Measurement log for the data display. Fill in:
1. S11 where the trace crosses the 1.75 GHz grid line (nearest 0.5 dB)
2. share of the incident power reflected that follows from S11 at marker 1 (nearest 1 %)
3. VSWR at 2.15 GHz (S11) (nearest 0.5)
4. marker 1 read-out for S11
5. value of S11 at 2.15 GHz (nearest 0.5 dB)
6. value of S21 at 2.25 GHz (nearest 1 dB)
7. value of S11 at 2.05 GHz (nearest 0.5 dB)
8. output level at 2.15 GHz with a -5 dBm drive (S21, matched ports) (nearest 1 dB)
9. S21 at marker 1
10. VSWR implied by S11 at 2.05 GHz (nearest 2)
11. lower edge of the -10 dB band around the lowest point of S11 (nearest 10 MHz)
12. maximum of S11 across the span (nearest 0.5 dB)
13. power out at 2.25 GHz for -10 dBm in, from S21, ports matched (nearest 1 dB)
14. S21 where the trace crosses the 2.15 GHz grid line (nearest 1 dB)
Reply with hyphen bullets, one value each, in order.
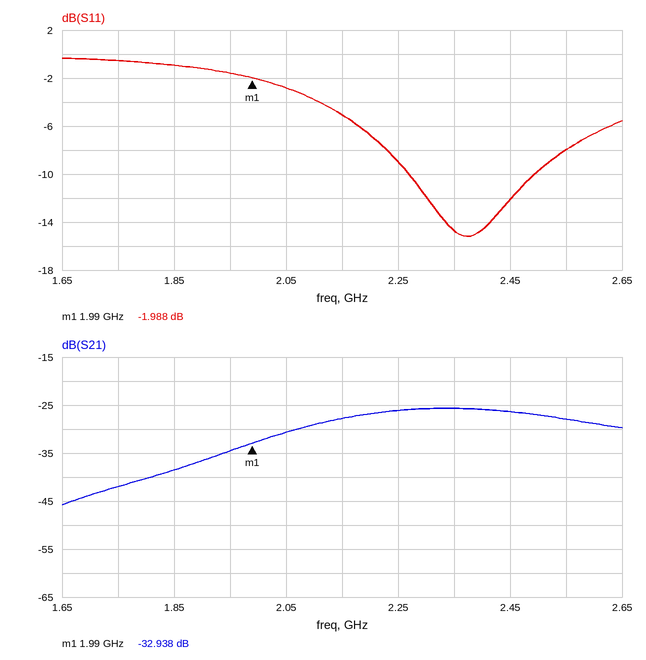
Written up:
- -0.5 dB
- 63 %
- 3.5
- -1.988 dB
- -5.0 dB
- -26 dB
- -3.0 dB
- -33 dBm
- -32.938 dB
- 6
- 2.27 GHz
- -0.5 dB
- -36 dBm
- -28 dB
